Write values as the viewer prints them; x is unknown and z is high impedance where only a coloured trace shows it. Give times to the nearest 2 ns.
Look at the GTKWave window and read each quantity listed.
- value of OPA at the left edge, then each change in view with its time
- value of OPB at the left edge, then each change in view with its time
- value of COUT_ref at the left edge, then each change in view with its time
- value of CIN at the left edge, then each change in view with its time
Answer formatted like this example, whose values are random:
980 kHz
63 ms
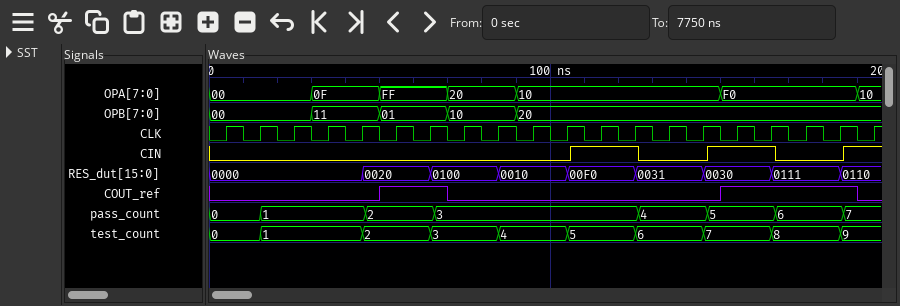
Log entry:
00, 0F at 30 ns, FF at 50 ns, 20 at 70 ns, 10 at 90 ns, F0 at 150 ns, 10 at 190 ns
00, 11 at 30 ns, 01 at 50 ns, 10 at 70 ns, 20 at 90 ns
0, 1 at 50 ns, 0 at 70 ns, 1 at 150 ns, 0 at 190 ns
0, 1 at 106 ns, 0 at 126 ns, 1 at 146 ns, 0 at 166 ns, 1 at 186 ns
